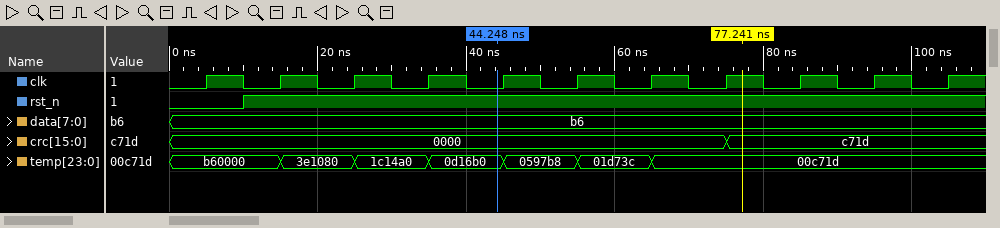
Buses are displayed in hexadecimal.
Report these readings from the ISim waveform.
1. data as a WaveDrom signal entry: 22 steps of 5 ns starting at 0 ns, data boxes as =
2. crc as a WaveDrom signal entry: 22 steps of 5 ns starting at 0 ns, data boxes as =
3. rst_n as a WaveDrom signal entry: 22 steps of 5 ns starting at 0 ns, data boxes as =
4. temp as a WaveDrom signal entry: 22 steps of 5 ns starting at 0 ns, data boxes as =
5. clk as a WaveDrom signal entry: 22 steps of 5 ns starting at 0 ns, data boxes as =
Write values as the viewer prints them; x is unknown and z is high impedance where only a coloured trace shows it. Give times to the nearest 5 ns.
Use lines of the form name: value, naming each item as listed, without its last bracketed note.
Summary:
data as a WaveDrom signal entry: 22 steps of 5 ns starting at 0 ns, data boxes as =: {name: 'data', wave: '=.....................', data: 'b6'}
crc as a WaveDrom signal entry: 22 steps of 5 ns starting at 0 ns, data boxes as =: {name: 'crc', wave: '=..............=......', data: '0000 c71d'}
rst_n as a WaveDrom signal entry: 22 steps of 5 ns starting at 0 ns, data boxes as =: {name: 'rst_n', wave: '0.1...................'}
temp as a WaveDrom signal entry: 22 steps of 5 ns starting at 0 ns, data boxes as =: {name: 'temp', wave: '=..=.=.=.=.=.=........', data: 'b60000 3e1080 1c14a0 0d16b0 0597b8 01d73c 00c71d'}
clk as a WaveDrom signal entry: 22 steps of 5 ns starting at 0 ns, data boxes as =: {name: 'clk', wave: '0101010101010101010101'}
